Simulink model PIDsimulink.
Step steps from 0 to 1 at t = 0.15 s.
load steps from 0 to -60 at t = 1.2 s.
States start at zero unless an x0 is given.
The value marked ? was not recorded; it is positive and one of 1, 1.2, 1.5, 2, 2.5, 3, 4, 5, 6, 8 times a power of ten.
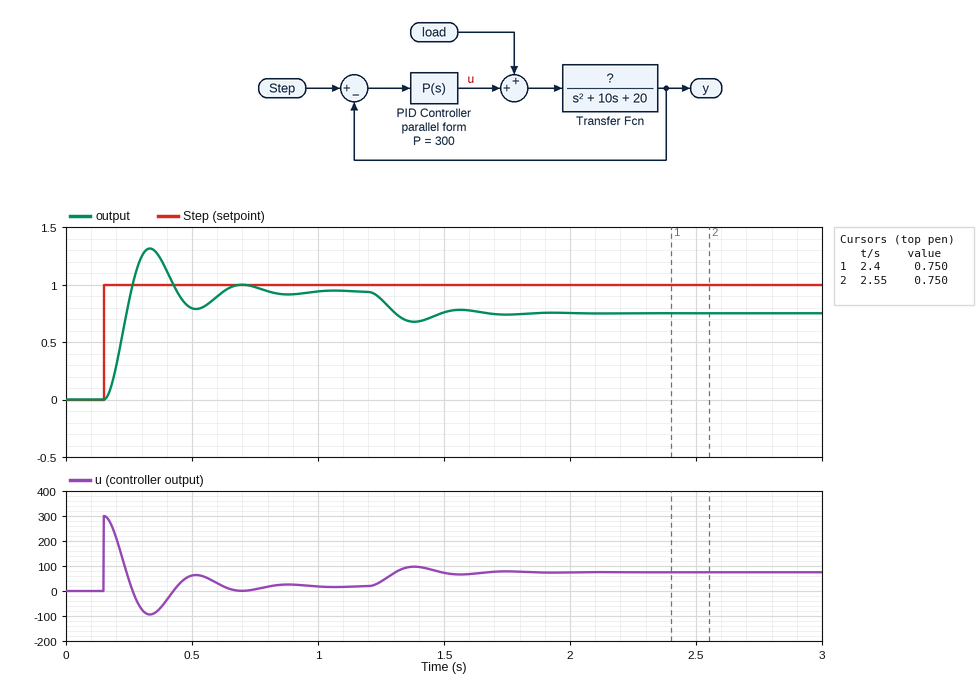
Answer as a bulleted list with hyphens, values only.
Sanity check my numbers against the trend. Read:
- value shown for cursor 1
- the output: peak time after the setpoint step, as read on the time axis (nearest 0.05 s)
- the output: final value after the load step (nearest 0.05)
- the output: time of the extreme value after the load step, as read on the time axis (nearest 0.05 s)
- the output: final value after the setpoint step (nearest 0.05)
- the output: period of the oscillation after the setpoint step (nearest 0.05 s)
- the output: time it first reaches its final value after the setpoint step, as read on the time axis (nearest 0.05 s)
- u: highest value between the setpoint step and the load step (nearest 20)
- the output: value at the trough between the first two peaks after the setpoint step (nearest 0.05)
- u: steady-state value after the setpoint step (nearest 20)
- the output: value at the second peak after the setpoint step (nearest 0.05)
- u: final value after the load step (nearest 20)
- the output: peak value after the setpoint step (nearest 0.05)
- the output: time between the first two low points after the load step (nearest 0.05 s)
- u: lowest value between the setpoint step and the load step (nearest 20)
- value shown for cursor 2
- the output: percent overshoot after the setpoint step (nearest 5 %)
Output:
- 0.750
- 0.35 s
- 0.75
- 1.40 s
- 0.95
- 0.35 s
- 0.25 s
- 300
- 0.80
- 20
- 1.00
- 80
- 1.30
- 0.35 s
- -100
- 0.750
- 40 %
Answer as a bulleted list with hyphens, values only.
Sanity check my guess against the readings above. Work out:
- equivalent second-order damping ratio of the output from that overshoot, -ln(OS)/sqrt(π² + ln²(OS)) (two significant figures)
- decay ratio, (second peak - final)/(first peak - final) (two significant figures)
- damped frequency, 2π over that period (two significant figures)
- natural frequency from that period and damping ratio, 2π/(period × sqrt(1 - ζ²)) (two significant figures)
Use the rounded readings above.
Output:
- 0.28
- 0.14
- 18 rad/s
- 19 rad/s
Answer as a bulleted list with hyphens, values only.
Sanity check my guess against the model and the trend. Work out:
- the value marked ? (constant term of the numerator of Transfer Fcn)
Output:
- 1
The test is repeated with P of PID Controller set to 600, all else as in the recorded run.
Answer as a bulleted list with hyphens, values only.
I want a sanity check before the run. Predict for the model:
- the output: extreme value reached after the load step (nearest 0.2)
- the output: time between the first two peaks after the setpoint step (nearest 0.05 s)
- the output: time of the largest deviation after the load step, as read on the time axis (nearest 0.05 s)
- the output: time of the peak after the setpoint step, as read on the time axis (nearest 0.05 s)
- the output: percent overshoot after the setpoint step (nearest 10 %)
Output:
- 0.8
- 0.25 s
- 1.35 s
- 0.30 s
- 50 %
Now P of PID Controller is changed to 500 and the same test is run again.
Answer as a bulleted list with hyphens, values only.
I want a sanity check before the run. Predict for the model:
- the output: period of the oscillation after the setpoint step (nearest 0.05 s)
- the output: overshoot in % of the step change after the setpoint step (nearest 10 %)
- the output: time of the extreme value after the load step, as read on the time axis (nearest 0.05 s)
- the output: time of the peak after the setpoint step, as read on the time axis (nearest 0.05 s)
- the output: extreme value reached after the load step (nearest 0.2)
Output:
- 0.30 s
- 50 %
- 1.35 s
- 0.30 s
- 0.8
